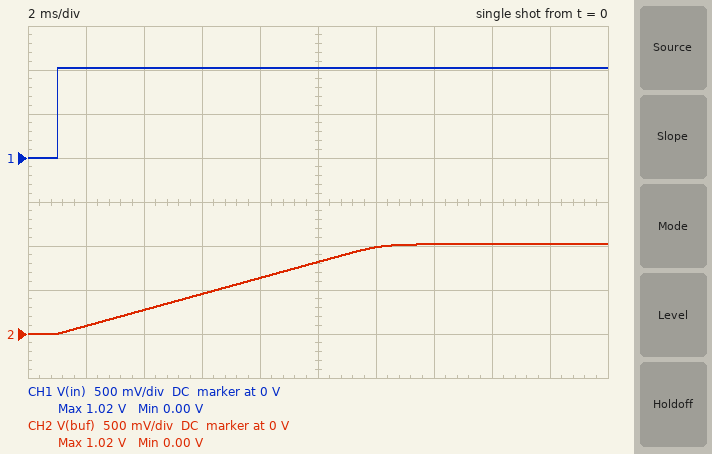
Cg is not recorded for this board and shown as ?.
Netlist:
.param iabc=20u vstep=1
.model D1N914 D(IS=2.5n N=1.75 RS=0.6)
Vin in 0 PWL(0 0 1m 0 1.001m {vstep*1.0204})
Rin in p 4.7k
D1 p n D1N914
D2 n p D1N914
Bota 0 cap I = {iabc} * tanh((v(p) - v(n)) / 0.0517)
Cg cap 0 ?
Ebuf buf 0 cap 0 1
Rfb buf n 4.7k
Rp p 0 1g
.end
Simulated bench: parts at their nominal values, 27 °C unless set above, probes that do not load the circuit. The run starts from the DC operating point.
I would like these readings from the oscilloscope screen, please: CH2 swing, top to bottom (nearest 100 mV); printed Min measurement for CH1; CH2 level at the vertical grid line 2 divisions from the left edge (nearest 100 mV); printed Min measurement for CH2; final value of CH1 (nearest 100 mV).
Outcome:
1.0 V
0.00 V
300 mV
0.00 V
1.0 V
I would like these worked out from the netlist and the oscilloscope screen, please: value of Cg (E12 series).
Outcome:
220 nF
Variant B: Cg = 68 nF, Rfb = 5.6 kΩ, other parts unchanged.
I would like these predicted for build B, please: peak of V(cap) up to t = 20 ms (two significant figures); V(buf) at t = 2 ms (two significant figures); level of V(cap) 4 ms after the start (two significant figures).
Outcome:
1.0 V
290 mV
880 mV
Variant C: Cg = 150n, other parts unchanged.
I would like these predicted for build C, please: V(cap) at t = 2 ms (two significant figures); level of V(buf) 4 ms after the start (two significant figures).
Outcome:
130 mV
400 mV
